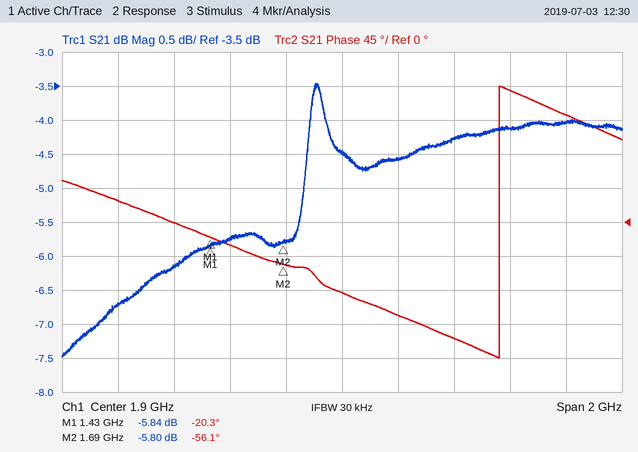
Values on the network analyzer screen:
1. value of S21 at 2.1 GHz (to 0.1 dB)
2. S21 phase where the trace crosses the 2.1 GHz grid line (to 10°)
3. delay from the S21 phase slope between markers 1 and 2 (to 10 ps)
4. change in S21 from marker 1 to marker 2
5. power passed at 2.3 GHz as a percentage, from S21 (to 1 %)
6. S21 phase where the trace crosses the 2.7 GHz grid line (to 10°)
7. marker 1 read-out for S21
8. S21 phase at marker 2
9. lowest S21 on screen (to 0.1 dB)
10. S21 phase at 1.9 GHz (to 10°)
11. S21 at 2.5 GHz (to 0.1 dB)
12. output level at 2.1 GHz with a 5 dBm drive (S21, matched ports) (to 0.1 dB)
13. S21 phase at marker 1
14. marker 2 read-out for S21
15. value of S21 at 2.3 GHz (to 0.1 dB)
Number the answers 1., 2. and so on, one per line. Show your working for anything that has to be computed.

1. -4.6 dB
2. -120°
3. −(-56.1° − (-20.3°))/(360° × 260 MHz) ≈ 382 ps, so 380 ps to the nearest 10 ps
4. -5.8 − (-5.84) = 0.04 dB
5. 10^(-4.3/10) ≈ 37 %
6. 140°
7. -5.84 dB
8. -56.1°
9. -7.5 dB
10. -90°
11. -4.1 dB
12. 5 dBm + (-4.6 dB) = 0.4 dBm
13. -20.3°
14. -5.80 dB
15. -4.3 dB
